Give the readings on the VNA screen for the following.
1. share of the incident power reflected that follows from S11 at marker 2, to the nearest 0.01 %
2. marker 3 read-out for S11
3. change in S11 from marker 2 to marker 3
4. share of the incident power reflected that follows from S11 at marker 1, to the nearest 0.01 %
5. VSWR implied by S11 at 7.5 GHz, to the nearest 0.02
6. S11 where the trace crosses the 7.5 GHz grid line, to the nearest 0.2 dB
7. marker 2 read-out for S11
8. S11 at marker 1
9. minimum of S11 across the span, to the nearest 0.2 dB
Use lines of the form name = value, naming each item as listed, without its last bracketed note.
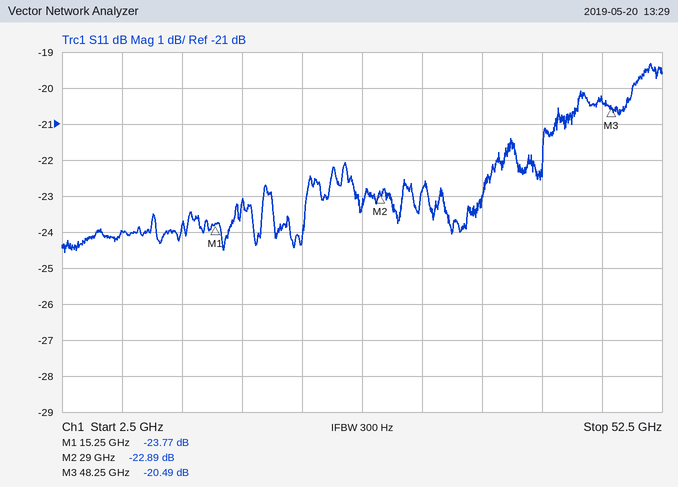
share of the incident power reflected that follows from S11 at marker 2, to the nearest 0.01 % = 0.51 %
marker 3 read-out for S11 = -20.49 dB
change in S11 from marker 2 to marker 3 = 2.40 dB
share of the incident power reflected that follows from S11 at marker 1, to the nearest 0.01 % = 0.42 %
VSWR implied by S11 at 7.5 GHz, to the nearest 0.02 = 1.14
S11 where the trace crosses the 7.5 GHz grid line, to the nearest 0.2 dB = -24.0 dB
marker 2 read-out for S11 = -22.89 dB
S11 at marker 1 = -23.77 dB
minimum of S11 across the span, to the nearest 0.2 dB = -24.6 dB
